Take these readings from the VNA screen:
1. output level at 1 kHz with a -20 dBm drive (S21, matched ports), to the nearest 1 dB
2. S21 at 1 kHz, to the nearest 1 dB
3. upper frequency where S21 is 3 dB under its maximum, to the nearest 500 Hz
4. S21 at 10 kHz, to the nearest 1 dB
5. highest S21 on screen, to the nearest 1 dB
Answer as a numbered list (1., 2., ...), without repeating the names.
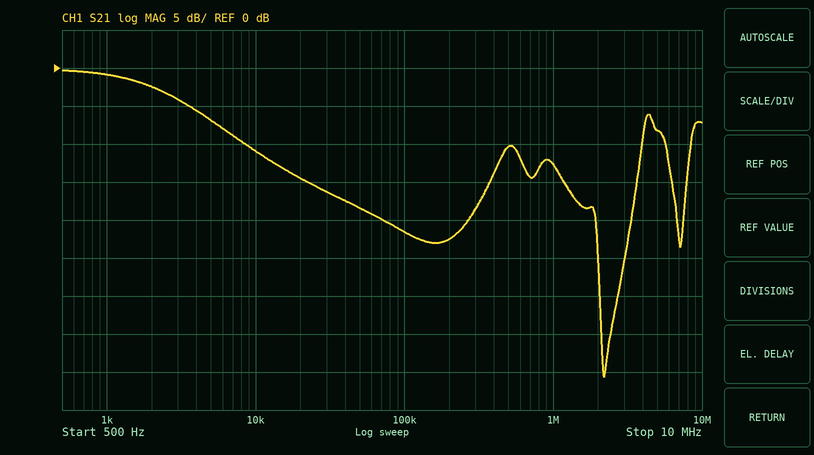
1. -21 dBm
2. -1 dB
3. 2.5 kHz
4. -11 dB
5. 0 dB
